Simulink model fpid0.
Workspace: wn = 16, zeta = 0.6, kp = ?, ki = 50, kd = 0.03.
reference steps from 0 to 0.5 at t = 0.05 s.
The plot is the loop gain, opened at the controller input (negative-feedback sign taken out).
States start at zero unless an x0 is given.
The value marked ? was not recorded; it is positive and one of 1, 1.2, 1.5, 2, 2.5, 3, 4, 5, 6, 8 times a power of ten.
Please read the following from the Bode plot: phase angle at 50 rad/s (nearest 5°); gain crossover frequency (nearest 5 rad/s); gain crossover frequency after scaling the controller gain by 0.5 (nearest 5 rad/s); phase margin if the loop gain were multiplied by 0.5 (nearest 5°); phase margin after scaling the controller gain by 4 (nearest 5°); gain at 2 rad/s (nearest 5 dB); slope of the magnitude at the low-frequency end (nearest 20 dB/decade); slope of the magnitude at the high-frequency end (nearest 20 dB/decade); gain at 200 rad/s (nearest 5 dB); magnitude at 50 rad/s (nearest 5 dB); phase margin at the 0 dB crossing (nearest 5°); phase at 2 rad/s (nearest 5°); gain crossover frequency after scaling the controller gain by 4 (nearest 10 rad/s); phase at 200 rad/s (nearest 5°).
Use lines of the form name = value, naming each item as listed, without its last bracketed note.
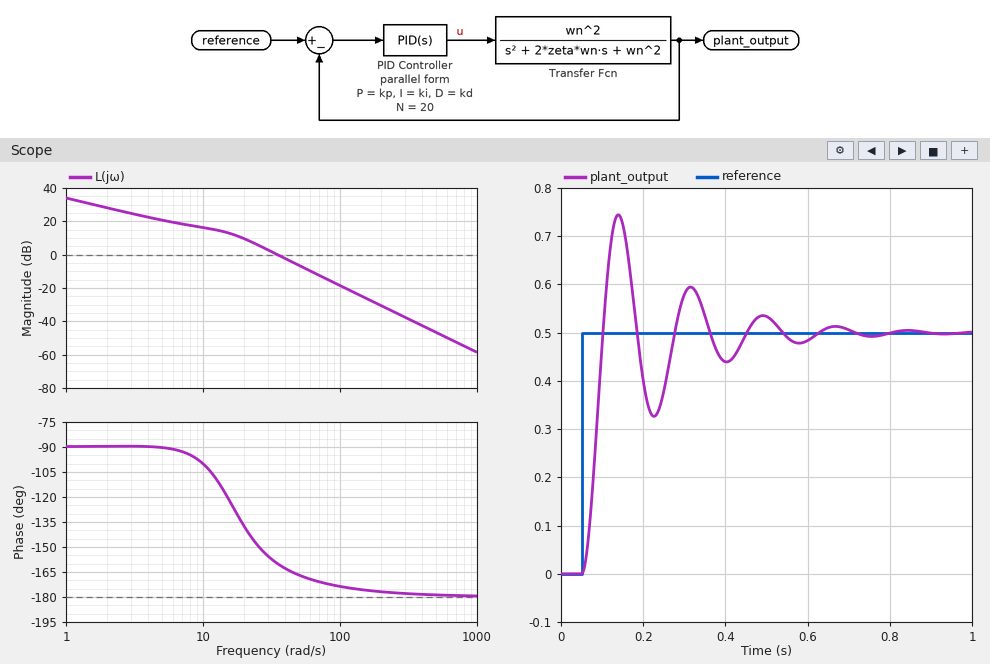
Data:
phase angle at 50 rad/s = -165°
gain crossover frequency = 35 rad/s
gain crossover frequency after scaling the controller gain by 0.5 = 25 rad/s
phase margin if the loop gain were multiplied by 0.5 = 30°
phase margin after scaling the controller gain by 4 = 10°
gain at 2 rad/s = 30 dB
slope of the magnitude at the low-frequency end = -20 dB/decade
slope of the magnitude at the high-frequency end = -40 dB/decade
gain at 200 rad/s = -30 dB
magnitude at 50 rad/s = -5 dB
phase margin at the 0 dB crossing = 20°
phase at 2 rad/s = -90°
gain crossover frequency after scaling the controller gain by 4 = 70 rad/s
phase at 200 rad/s = -175°
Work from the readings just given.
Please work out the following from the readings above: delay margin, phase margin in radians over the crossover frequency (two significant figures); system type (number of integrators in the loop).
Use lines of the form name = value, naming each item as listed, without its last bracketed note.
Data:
delay margin, phase margin in radians over the crossover frequency = 0.0100 s
system type = 1
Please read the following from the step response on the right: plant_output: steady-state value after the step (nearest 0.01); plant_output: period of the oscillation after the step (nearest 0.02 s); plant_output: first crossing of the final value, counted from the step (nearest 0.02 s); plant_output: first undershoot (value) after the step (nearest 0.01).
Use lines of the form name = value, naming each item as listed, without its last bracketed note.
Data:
plant_output: steady-state value after the step = 0.50
plant_output: period of the oscillation after the step = 0.18 s
plant_output: first crossing of the final value, counted from the step = 0.06 s
plant_output: first undershoot (value) after the step = 0.33
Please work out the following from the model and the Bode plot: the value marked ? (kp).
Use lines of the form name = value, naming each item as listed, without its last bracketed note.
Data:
the value marked ? = 4
